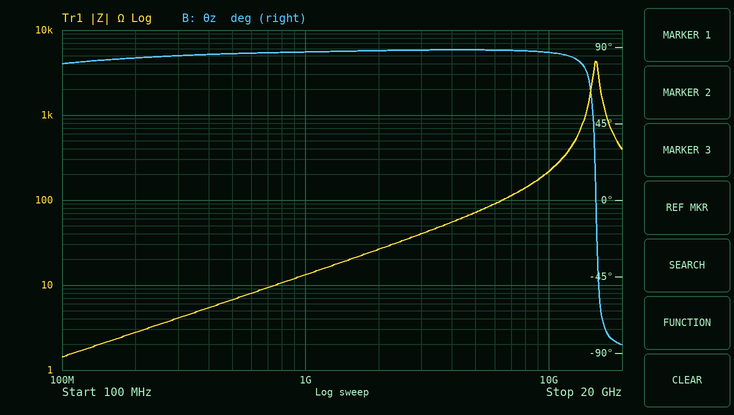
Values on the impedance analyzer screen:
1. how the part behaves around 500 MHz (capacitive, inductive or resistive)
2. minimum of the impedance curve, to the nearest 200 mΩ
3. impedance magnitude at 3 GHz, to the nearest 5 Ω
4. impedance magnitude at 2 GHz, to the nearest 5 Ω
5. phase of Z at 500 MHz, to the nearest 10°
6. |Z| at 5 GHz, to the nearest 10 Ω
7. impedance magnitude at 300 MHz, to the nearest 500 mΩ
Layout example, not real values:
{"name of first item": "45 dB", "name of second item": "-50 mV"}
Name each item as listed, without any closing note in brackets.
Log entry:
{"how the part behaves around 500 MHz": "inductive", "minimum of the impedance curve, to the nearest 200 mΩ": "1.4 Ω", "impedance magnitude at 3 GHz, to the nearest 5 Ω": "40 Ω", "impedance magnitude at 2 GHz, to the nearest 5 Ω": "25 Ω", "phase of Z at 500 MHz, to the nearest 10°": "90°", "|Z| at 5 GHz, to the nearest 10 Ω": "70 Ω", "impedance magnitude at 300 MHz, to the nearest 500 mΩ": "4.0 Ω"}
